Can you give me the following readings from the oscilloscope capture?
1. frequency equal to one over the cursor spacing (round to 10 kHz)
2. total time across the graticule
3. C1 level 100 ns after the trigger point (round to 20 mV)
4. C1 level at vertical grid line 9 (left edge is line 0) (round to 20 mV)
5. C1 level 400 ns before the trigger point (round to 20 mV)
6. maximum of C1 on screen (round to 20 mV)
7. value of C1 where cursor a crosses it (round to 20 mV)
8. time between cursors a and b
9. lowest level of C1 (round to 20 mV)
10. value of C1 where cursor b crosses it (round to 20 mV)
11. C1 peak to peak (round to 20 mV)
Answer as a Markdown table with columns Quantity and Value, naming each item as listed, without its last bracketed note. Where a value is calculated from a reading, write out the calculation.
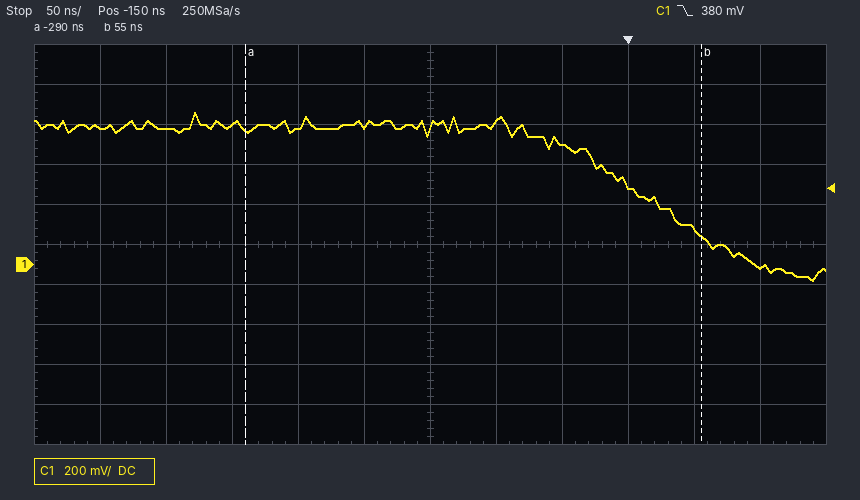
| Quantity | Value |
|---|---|
| frequency equal to one over the cursor spacing | 1 / 345 ns ≈ 2.90 MHz |
| total time across the graticule | 600 ns |
| C1 level 100 ns after the trigger point | -20 mV |
| C1 level at vertical grid line 9 (left edge is line 0) | 400 mV |
| C1 level 400 ns before the trigger point | 680 mV |
| maximum of C1 on screen | 760 mV |
| value of C1 where cursor a crosses it | 680 mV |
| time between cursors a and b | 55 ns − (-290 ns) = 345 ns |
| lowest level of C1 | -80 mV |
| value of C1 where cursor b crosses it | 140 mV |
| C1 peak to peak | 760 mV − (-80 mV) = 840 mV |
